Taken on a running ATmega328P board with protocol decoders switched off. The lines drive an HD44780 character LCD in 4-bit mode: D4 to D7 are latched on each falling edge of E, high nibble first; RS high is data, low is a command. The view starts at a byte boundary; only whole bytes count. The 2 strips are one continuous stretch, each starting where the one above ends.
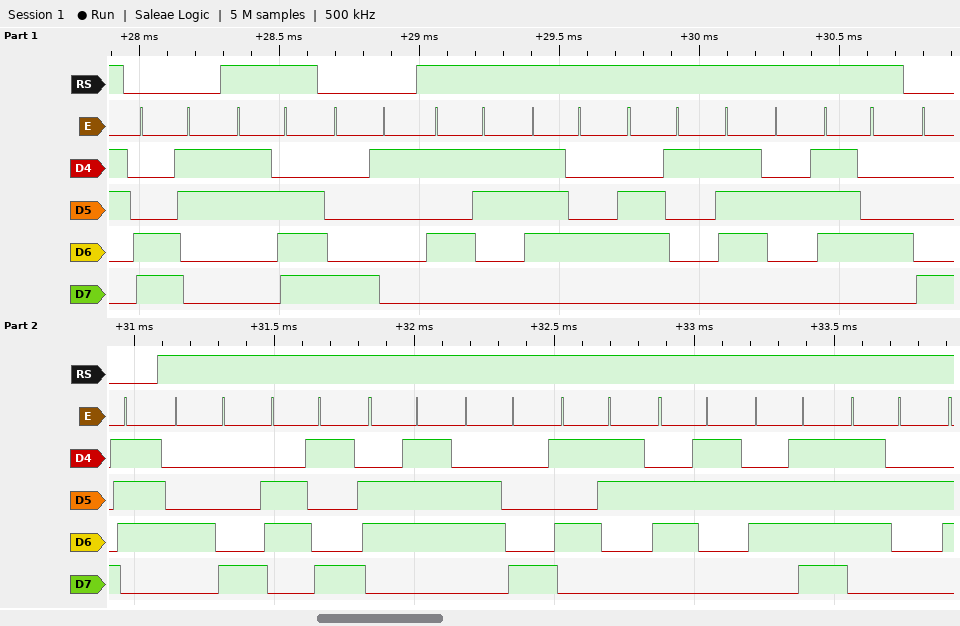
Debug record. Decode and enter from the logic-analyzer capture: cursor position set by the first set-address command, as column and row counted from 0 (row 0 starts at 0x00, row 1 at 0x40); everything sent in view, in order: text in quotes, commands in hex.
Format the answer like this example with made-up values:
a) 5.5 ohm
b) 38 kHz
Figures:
a) column 3, row 1
b) 0xC3 ">" 0x81 "Start" 0x87 "HighScor"
